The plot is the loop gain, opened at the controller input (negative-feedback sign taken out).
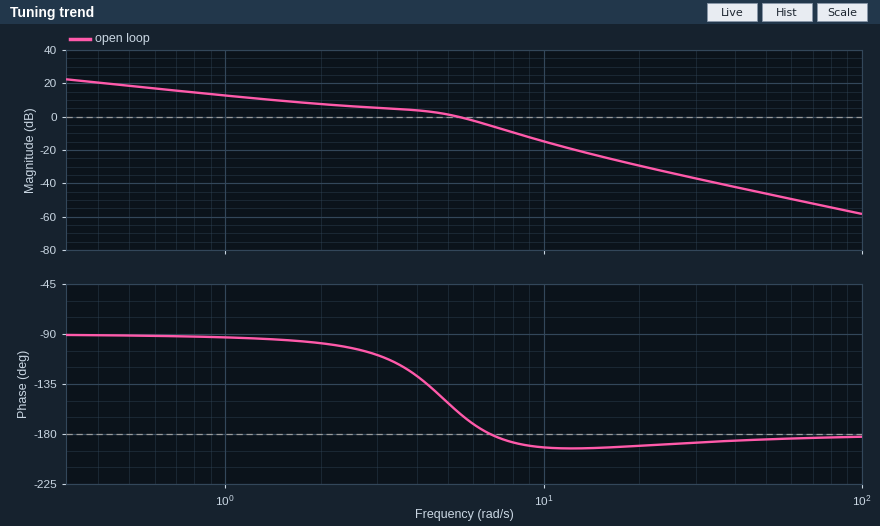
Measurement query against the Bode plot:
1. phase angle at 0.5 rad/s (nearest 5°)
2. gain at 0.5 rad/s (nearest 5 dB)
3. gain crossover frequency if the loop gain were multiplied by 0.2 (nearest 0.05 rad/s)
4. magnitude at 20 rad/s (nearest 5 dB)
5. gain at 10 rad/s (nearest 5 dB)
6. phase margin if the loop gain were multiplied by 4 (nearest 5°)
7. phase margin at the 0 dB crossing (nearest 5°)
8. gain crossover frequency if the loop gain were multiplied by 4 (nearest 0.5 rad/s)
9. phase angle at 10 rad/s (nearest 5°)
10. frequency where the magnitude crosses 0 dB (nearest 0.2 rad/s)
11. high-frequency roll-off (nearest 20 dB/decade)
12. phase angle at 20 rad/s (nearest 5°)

-90°
20 dB
0.85 rad/s
-30 dB
-15 dB
-10°
20°
9.0 rad/s
-190°
5.4 rad/s
-40 dB/decade
-190°
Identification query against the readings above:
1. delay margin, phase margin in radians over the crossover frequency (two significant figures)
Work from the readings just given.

0.065 s
